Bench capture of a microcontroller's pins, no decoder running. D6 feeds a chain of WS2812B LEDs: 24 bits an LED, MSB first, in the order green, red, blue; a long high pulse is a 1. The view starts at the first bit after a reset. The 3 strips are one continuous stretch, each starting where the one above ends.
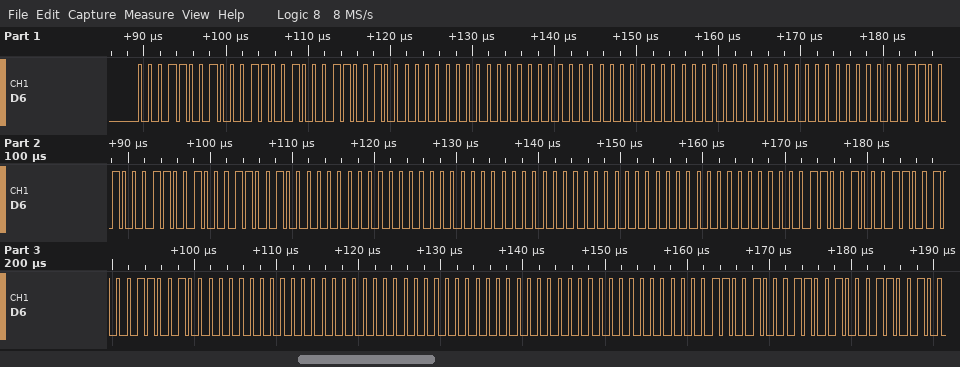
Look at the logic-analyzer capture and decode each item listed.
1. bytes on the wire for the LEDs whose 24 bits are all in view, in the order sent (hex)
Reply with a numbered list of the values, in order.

1. 19 19 19 00 00 00 00 00 00 19 19 19 00 00 00 00 00 00 19 19 19 00 00 00 00 00 00 19 19 19
